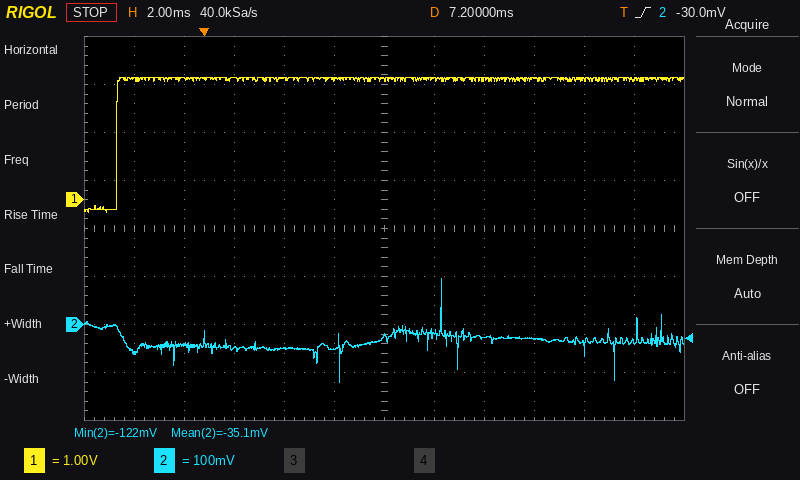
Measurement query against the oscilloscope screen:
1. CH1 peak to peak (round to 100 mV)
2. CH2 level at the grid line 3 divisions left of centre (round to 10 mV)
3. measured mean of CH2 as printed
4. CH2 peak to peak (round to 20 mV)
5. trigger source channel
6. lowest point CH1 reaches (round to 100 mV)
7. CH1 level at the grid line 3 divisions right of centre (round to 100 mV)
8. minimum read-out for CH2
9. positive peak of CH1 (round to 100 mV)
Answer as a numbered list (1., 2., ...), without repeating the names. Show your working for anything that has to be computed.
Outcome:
1. 2.5 V − (-300 mV) = 2.8 V
2. -50 mV
3. -35.1 mV
4. 220 mV
5. CH2
6. -300 mV
7. 2.5 V
8. -122 mV
9. 2.5 V
